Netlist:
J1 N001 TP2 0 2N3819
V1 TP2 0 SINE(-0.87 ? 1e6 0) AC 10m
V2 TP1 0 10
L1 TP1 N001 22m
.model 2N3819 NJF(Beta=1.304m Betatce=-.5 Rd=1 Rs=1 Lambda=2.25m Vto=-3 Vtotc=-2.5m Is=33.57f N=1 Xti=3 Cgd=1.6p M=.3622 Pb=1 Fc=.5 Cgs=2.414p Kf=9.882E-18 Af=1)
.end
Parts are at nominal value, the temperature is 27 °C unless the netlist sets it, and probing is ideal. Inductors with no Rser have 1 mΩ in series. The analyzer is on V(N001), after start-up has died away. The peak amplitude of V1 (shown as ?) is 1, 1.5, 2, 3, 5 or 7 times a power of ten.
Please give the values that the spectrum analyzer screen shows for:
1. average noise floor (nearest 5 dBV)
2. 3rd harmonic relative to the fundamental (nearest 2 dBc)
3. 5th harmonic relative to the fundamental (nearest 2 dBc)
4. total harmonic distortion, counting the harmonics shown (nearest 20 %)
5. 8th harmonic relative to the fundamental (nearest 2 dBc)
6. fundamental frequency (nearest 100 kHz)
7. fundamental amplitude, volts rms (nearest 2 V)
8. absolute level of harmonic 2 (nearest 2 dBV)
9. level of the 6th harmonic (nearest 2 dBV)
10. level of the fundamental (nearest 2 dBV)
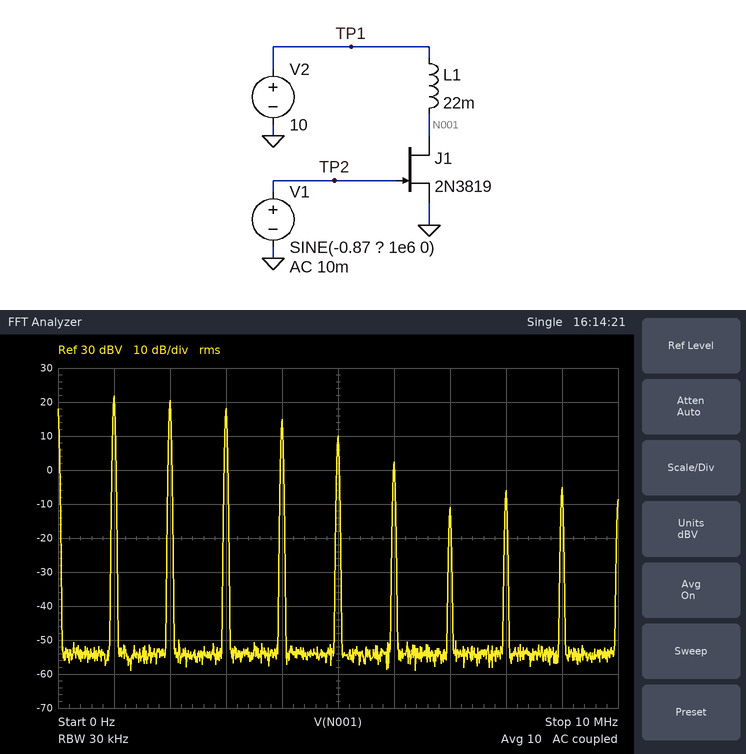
-55 dBV
-4 dBc
-12 dBc
120 %
-28 dBc
1.0 MHz
12 V
20 dBV
2 dBV
22 dBV
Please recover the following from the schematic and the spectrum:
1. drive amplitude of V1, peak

500 mV
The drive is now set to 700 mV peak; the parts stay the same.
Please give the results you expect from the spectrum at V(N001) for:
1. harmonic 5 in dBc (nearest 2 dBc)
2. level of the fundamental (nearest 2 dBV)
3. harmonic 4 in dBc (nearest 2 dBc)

-8 dBc
22 dBV
-6 dBc
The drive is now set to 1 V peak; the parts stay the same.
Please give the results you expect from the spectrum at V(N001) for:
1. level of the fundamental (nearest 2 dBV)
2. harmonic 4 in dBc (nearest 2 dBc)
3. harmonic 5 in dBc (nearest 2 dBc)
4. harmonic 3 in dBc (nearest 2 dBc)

22 dBV
-4 dBc
-6 dBc
-2 dBc
